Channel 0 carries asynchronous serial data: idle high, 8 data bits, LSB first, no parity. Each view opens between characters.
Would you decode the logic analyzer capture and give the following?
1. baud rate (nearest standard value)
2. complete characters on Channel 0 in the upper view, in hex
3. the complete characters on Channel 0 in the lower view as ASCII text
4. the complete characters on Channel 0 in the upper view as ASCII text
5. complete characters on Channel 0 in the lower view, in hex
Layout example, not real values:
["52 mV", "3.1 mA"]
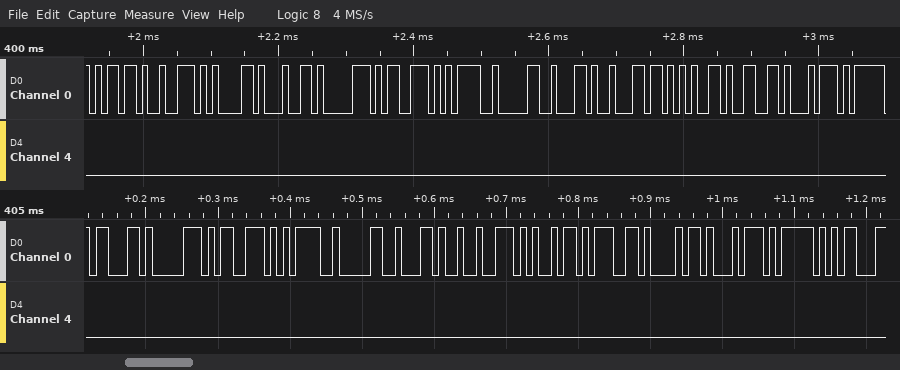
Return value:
["115200 baud", "6D, 72, 61, 64, 70, 73, 3D, 30, 2C, 6C, 65, 66, 74", "\"cps=0,right_\"", "\"mradps=0,left\"", "63, 70, 73, 3D, 30, 2C, 72, 69, 67, 68, 74, 5F"]
